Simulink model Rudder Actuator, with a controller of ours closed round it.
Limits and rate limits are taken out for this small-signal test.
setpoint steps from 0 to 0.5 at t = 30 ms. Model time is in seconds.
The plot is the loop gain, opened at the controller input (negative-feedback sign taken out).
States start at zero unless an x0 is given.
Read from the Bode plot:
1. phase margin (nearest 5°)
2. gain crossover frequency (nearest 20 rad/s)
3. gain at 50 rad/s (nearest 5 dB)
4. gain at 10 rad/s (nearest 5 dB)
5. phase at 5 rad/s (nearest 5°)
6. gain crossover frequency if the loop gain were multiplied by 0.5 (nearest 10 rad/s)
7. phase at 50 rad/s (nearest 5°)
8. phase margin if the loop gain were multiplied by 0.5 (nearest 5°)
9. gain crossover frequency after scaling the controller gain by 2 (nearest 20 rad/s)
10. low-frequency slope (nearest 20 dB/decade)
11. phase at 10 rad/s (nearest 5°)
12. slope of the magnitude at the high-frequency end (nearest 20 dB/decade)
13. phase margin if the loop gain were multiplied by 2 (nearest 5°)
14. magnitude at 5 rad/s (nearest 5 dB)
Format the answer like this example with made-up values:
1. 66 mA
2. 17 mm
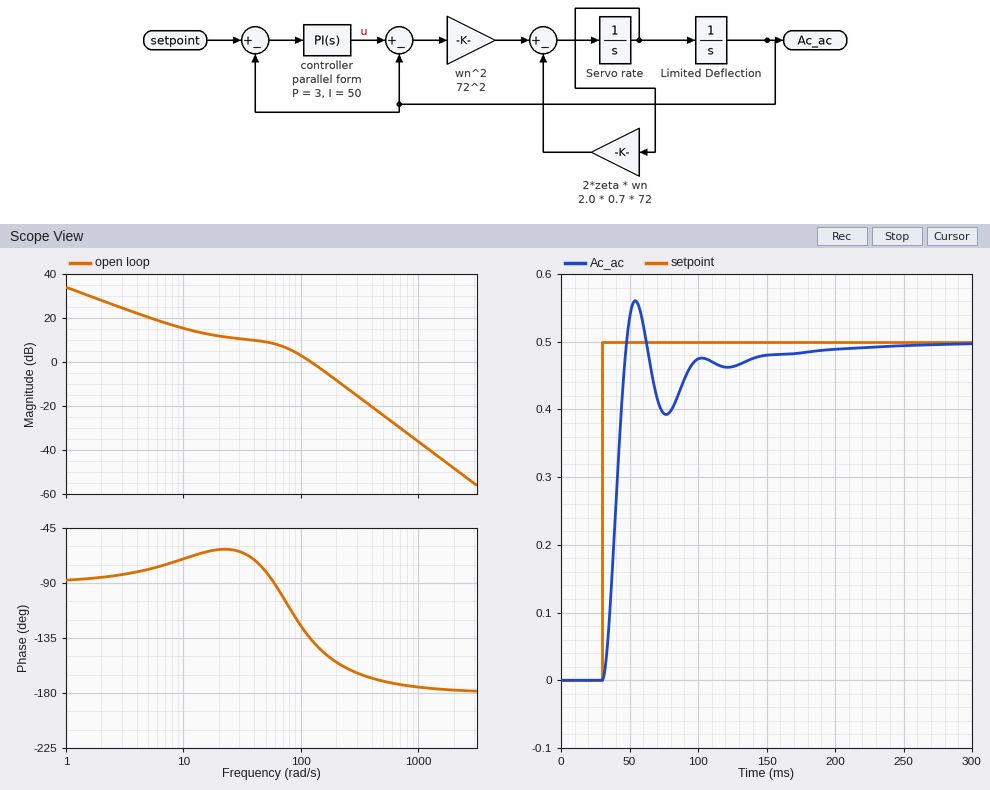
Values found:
1. 45°
2. 120 rad/s
3. 10 dB
4. 15 dB
5. -80°
6. 80 rad/s
7. -80°
8. 70°
9. 180 rad/s
10. -20 dB/decade
11. -70°
12. -40 dB/decade
13. 30°
14. 20 dB
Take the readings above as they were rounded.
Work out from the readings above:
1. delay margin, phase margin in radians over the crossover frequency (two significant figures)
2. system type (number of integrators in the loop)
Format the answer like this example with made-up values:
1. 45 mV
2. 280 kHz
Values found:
1. 0.0065 s
2. 1
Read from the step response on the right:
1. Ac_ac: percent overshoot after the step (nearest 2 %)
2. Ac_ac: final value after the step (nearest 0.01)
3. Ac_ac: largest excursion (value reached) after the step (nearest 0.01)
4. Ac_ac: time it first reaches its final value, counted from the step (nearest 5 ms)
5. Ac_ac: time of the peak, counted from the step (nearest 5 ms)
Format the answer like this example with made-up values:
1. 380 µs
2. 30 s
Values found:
1. 12 %
2. 0.50
3. 0.56
4. 20 ms
5. 25 ms
